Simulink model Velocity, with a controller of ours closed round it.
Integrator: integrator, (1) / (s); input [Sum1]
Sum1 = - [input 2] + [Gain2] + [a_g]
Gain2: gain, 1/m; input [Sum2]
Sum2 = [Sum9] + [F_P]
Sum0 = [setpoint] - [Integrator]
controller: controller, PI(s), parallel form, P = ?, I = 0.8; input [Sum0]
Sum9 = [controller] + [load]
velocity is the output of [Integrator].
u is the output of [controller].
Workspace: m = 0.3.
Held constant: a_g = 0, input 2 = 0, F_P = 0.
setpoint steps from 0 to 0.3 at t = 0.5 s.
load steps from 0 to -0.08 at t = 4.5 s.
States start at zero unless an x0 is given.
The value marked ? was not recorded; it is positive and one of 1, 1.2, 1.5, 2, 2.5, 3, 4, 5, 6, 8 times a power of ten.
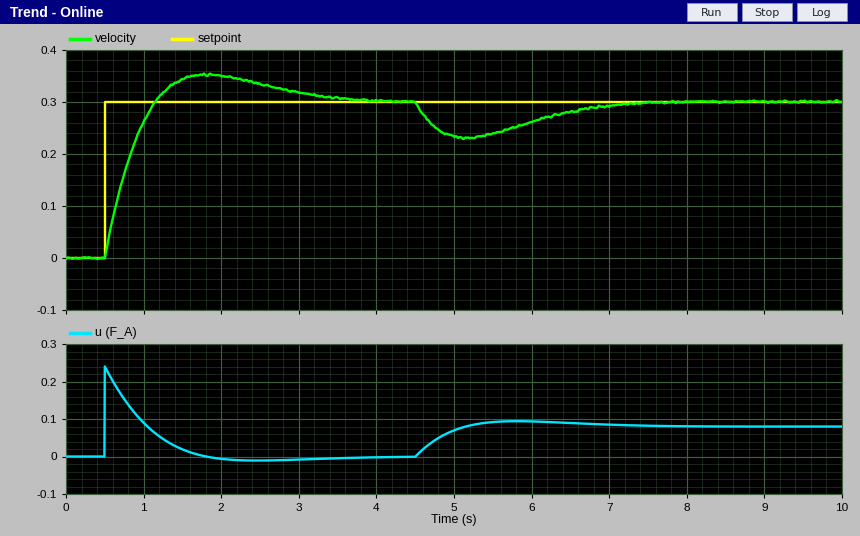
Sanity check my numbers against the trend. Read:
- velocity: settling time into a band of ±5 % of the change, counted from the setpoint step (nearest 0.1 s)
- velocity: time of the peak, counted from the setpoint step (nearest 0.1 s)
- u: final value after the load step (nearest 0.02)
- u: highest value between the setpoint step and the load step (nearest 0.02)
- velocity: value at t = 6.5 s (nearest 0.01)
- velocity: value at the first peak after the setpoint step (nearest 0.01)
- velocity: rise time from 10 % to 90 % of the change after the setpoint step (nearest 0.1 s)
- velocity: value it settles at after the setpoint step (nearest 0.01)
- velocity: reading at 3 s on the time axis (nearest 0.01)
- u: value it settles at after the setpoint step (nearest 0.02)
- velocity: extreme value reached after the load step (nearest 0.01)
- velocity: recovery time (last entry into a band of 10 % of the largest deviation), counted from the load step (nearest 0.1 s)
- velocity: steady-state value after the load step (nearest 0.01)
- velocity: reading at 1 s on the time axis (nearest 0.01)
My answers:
2.6 s
1.3 s
0.08
0.24
0.28
0.35
0.5 s
0.30
0.32
0.00
0.23
2.5 s
0.30
0.26
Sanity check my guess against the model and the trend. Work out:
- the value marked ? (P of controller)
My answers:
0.8
